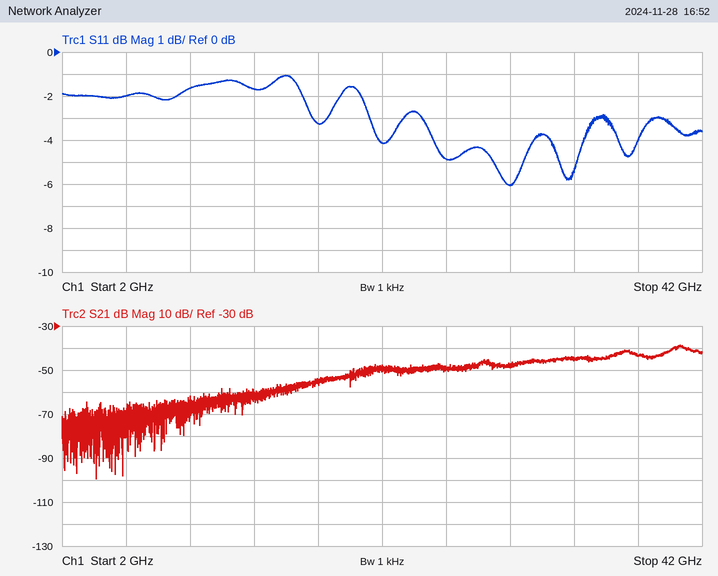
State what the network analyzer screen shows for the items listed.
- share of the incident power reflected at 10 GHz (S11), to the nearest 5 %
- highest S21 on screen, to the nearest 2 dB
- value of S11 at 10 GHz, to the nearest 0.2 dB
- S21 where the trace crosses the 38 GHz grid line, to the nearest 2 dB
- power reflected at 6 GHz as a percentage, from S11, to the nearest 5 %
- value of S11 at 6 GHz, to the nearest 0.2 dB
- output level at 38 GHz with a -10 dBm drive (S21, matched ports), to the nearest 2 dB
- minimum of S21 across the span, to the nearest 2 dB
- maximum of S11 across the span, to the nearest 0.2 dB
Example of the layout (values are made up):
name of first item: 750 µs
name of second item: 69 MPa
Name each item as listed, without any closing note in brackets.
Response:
share of the incident power reflected at 10 GHz (S11), to the nearest 5 %: 70 %
highest S21 on screen, to the nearest 2 dB: -38 dB
value of S11 at 10 GHz, to the nearest 0.2 dB: -1.6 dB
S21 where the trace crosses the 38 GHz grid line, to the nearest 2 dB: -44 dB
power reflected at 6 GHz as a percentage, from S11, to the nearest 5 %: 65 %
value of S11 at 6 GHz, to the nearest 0.2 dB: -2.0 dB
output level at 38 GHz with a -10 dBm drive (S21, matched ports), to the nearest 2 dB: -54 dBm
minimum of S21 across the span, to the nearest 2 dB: -100 dB
maximum of S11 across the span, to the nearest 0.2 dB: -1.0 dB
